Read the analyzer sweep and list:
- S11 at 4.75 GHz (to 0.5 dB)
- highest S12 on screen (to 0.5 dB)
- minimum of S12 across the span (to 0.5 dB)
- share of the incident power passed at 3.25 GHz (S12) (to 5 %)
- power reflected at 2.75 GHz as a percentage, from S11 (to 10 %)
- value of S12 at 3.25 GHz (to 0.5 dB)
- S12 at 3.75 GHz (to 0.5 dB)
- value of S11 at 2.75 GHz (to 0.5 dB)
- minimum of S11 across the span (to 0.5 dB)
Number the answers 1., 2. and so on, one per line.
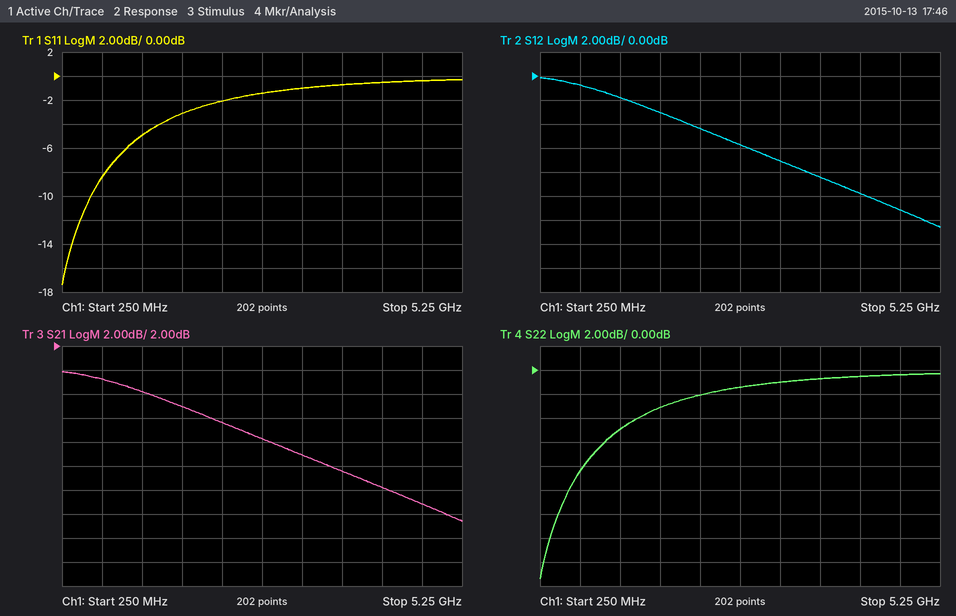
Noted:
1. -0.5 dB
2. 0.0 dB
3. -12.5 dB
4. 20 %
5. 70 %
6. -7.0 dB
7. -8.5 dB
8. -1.5 dB
9. -17.5 dB
